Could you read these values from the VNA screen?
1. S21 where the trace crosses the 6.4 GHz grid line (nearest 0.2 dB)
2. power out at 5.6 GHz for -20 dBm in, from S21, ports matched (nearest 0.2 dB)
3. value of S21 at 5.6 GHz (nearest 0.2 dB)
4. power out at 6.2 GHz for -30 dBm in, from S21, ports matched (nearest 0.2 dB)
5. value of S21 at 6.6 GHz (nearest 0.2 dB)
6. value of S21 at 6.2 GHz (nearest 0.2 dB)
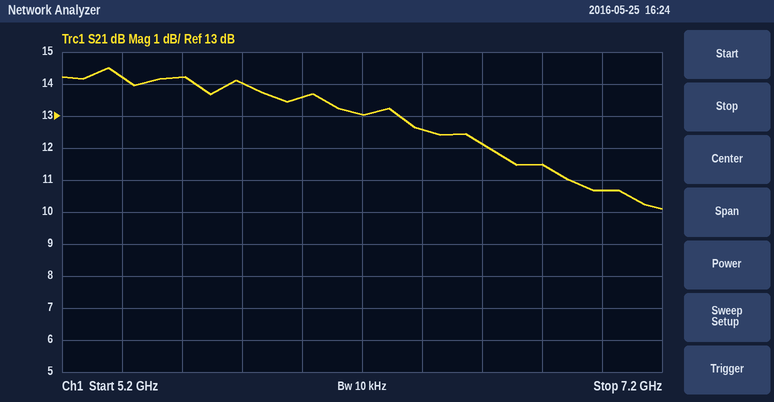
12.6 dB
-5.8 dBm
14.2 dB
-17.0 dBm
12.2 dB
13.0 dB
